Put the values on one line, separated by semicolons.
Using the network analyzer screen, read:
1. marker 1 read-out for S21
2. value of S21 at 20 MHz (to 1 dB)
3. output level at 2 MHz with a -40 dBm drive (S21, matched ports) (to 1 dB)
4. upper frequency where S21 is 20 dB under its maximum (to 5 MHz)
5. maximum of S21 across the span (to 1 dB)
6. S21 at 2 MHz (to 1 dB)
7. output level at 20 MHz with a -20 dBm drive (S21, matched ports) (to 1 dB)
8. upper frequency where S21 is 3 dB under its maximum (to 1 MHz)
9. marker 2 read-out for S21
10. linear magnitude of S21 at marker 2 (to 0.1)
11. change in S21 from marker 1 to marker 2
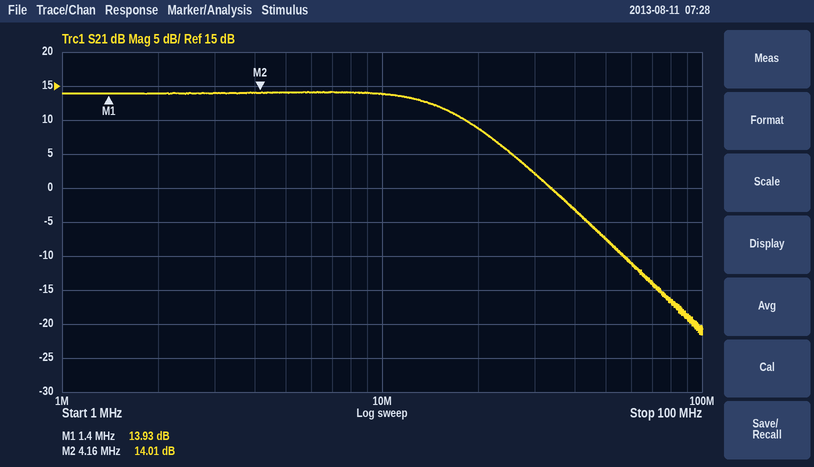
13.93 dB; 9 dB; -26 dBm; 45 MHz; 14 dB; 14 dB; -11 dBm; 16 MHz; 14.01 dB; 5.0; 0.08 dB
